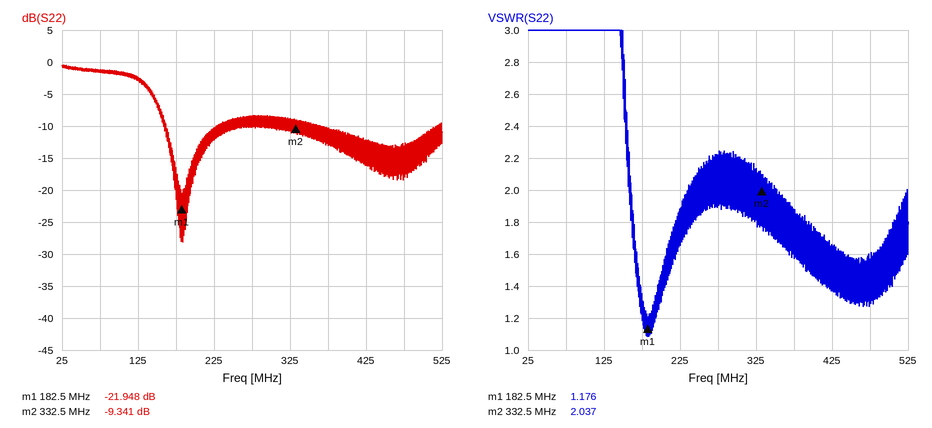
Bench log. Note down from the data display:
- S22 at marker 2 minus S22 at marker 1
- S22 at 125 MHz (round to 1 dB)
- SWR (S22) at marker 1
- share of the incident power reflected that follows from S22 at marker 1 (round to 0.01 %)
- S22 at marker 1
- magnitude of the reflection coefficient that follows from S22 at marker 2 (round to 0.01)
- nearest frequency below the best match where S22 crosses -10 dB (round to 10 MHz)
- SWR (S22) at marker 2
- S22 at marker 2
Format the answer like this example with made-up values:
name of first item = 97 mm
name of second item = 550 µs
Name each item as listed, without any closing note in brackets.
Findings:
S22 at marker 2 minus S22 at marker 1 = 12.607 dB
S22 at 125 MHz = -3 dB
SWR (S22) at marker 1 = 1.176
share of the incident power reflected that follows from S22 at marker 1 = 0.64 %
S22 at marker 1 = -21.948 dB
magnitude of the reflection coefficient that follows from S22 at marker 2 = 0.34
nearest frequency below the best match where S22 crosses -10 dB = 160 MHz
SWR (S22) at marker 2 = 2.037
S22 at marker 2 = -9.341 dB
